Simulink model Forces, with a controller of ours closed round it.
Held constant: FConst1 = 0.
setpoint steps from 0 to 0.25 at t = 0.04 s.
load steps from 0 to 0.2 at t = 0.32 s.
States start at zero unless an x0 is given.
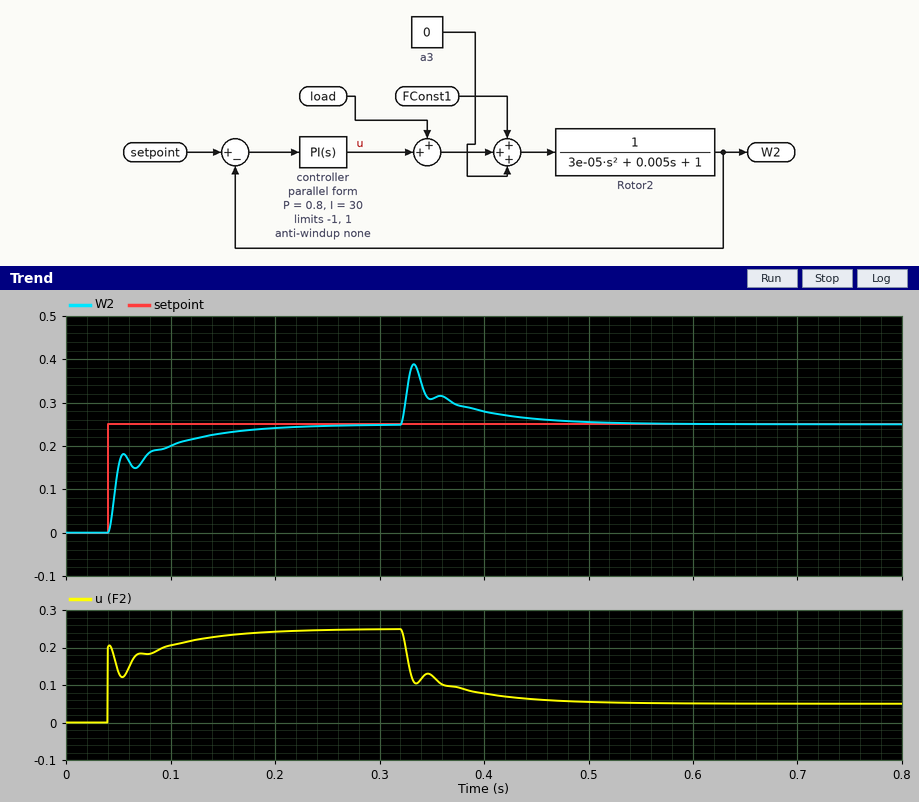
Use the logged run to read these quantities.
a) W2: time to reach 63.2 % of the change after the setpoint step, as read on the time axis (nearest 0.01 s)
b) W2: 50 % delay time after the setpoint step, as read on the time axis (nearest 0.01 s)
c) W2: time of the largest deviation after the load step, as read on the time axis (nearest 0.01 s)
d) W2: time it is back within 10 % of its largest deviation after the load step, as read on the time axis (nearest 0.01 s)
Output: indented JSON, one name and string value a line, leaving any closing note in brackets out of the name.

{
  "W2: time to reach 63.2 % of the change after the setpoint step, as read on the time axis": "0.05 s",
  "W2: 50 % delay time after the setpoint step, as read on the time axis": "0.05 s",
  "W2: time of the largest deviation after the load step, as read on the time axis": "0.33 s",
  "W2: time it is back within 10 % of its largest deviation after the load step, as read on the time axis": "0.44 s"
}
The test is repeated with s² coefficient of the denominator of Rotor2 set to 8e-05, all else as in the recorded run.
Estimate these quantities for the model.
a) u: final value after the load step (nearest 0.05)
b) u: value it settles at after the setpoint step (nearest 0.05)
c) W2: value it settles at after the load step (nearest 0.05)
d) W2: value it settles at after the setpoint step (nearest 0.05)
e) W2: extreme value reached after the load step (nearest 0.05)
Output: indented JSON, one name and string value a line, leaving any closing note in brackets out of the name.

{
  "u: final value after the load step": "0.05",
  "u: value it settles at after the setpoint step": "0.25",
  "W2: value it settles at after the load step": "0.25",
  "W2: value it settles at after the setpoint step": "0.25",
  "W2: extreme value reached after the load step": "0.40"
}
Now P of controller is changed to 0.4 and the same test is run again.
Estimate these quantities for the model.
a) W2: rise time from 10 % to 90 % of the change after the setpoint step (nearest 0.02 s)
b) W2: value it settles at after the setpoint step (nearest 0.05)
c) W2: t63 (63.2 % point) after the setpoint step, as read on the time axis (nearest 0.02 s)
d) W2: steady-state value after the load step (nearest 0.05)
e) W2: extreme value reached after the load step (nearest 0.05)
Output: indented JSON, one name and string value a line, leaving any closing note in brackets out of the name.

{
  "W2: rise time from 10 % to 90 % of the change after the setpoint step": "0.08 s",
  "W2: value it settles at after the setpoint step": "0.25",
  "W2: t63 (63.2 % point) after the setpoint step, as read on the time axis": "0.08 s",
  "W2: steady-state value after the load step": "0.25",
  "W2: extreme value reached after the load step": "0.40"
}
